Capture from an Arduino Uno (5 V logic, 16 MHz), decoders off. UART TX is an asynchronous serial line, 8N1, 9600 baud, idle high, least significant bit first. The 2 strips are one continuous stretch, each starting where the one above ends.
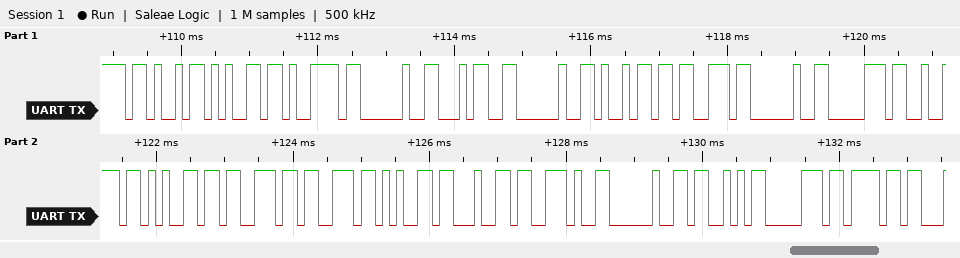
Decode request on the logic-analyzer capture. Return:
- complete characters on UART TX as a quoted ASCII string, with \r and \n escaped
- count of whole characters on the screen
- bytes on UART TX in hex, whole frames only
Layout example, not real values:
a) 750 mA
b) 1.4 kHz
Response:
a) "Key 4 is pressed. Spo"
b) 21
c) 0x4B 0x65 0x79 0x20 0x34 0x20 0x69 0x73 0x20 0x70 0x72 0x65 0x73 0x73 0x65 0x64 0x2E 0x20 0x53 0x70 0x6F
